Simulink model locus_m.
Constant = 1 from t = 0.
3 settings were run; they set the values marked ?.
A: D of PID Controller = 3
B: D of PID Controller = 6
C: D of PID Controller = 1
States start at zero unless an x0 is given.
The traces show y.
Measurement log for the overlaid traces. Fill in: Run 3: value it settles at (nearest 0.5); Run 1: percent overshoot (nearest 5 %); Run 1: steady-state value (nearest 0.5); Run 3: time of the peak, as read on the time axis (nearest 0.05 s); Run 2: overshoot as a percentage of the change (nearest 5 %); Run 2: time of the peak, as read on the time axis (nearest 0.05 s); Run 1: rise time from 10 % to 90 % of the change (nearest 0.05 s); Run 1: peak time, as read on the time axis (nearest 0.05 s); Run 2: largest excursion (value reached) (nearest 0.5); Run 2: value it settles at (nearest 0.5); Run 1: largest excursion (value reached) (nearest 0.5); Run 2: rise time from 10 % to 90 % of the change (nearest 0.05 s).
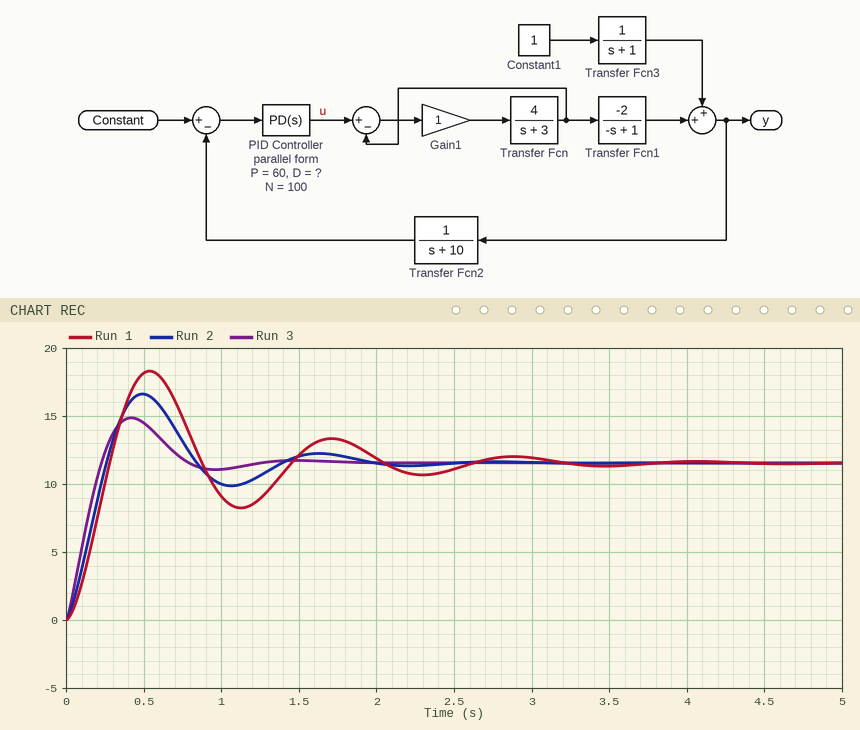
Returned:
11.5
60 %
11.5
0.40 s
45 %
0.50 s
0.20 s
0.55 s
16.5
11.5
18.5
0.20 s
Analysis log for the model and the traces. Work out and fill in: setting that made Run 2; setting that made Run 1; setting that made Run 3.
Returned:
A
C
B
